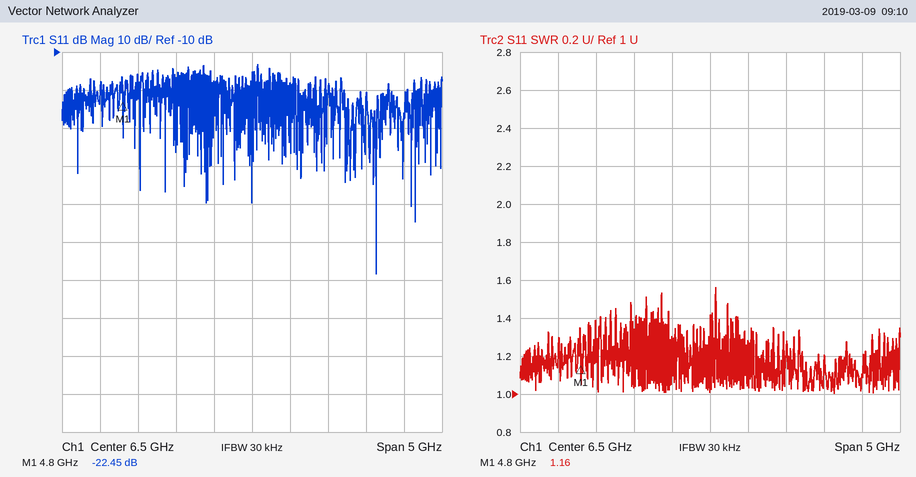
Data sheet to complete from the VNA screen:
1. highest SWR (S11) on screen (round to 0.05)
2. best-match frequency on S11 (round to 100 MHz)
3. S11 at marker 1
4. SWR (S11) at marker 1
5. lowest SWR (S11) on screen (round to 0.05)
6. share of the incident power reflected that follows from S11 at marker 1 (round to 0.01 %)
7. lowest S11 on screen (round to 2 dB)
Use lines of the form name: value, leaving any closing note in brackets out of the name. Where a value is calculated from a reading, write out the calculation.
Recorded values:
highest SWR (S11) on screen: 1.55
best-match frequency on S11: 8.1 GHz
S11 at marker 1: -22.45 dB
SWR (S11) at marker 1: 1.16
lowest SWR (S11) on screen: 1.00
share of the incident power reflected that follows from S11 at marker 1: 10^(-22.45/10) ≈ 0.57 %
lowest S11 on screen: -68 dB
